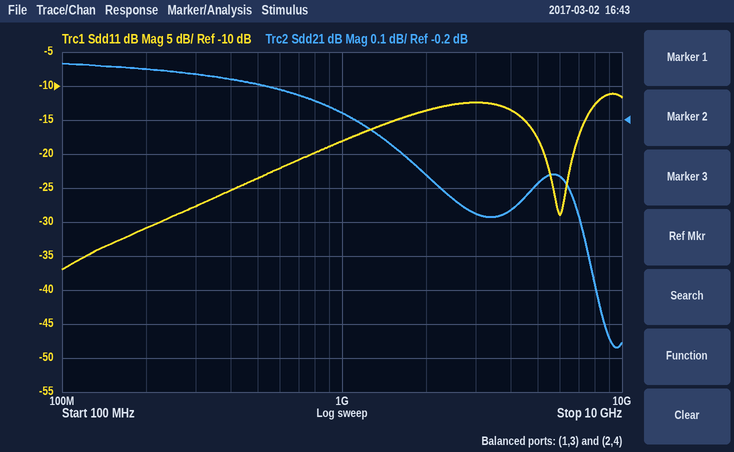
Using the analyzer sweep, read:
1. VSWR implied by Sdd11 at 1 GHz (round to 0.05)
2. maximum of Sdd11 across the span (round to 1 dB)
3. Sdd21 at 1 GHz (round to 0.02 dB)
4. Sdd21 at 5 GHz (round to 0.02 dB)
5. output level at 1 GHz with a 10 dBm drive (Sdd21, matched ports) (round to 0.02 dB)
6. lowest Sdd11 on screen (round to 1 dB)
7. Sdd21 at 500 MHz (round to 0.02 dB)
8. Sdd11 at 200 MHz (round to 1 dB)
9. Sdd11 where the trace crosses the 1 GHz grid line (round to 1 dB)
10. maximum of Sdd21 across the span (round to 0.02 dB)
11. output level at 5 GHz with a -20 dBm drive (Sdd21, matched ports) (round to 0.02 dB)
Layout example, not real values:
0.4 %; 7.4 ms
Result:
1.30; -11 dB; -0.18 dB; -0.38 dB; 9.82 dBm; -37 dB; -0.10 dB; -31 dB; -18 dB; -0.04 dB; -20.38 dBm
